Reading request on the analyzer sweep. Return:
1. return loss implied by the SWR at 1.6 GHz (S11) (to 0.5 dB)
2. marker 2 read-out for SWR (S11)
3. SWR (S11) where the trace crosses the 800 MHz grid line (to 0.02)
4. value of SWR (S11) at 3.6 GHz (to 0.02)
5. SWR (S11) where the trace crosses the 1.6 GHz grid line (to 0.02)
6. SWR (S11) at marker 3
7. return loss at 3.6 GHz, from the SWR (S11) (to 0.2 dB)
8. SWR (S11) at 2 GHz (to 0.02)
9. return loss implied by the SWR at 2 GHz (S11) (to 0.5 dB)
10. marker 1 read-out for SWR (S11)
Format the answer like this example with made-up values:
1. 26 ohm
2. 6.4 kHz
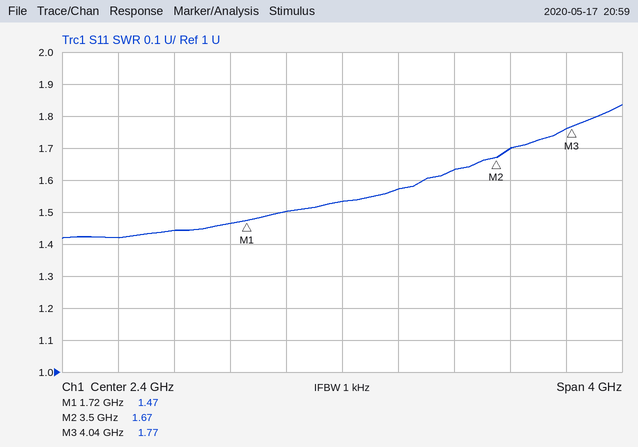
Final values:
1. 14.5 dB
2. 1.67
3. 1.42
4. 1.70
5. 1.46
6. 1.77
7. 11.8 dB
8. 1.50
9. 14.0 dB
10. 1.47
